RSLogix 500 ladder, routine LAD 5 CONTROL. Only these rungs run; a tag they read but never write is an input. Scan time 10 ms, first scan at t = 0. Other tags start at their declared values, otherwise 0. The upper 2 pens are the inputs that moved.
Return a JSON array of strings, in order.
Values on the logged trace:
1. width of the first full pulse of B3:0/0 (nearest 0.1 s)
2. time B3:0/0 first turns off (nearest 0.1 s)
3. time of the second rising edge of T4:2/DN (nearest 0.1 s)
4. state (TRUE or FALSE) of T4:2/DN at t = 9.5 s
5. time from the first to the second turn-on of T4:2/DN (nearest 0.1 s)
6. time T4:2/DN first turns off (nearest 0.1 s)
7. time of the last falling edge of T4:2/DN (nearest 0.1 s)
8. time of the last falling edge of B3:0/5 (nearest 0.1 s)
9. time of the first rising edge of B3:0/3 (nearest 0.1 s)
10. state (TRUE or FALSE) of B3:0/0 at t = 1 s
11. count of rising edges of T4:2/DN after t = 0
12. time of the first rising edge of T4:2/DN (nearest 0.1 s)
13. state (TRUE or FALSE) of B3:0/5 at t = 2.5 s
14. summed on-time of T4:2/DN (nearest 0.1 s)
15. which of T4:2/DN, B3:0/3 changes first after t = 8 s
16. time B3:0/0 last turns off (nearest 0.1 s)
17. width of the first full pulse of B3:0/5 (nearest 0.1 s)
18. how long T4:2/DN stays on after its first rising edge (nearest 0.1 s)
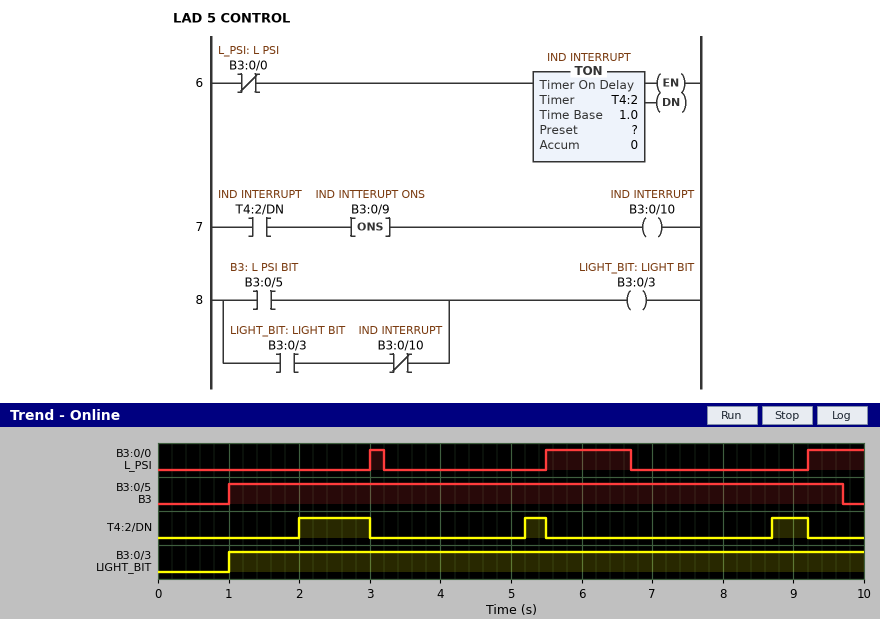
["0.2 s", "3.2 s", "5.2 s", "FALSE", "3.2 s", "3.0 s", "9.2 s", "9.7 s", "1.0 s", "FALSE", "3", "2.0 s", "TRUE", "1.8 s", "T4:2/DN", "6.7 s", "8.7 s", "1.0 s"]
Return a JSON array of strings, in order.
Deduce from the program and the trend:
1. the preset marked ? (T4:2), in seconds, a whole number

["2 s"]
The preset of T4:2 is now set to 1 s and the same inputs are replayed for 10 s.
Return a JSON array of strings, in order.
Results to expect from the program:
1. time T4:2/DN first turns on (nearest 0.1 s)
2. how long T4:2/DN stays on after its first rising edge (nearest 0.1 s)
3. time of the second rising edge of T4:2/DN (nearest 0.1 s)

["1.0 s", "2.0 s", "4.2 s"]
